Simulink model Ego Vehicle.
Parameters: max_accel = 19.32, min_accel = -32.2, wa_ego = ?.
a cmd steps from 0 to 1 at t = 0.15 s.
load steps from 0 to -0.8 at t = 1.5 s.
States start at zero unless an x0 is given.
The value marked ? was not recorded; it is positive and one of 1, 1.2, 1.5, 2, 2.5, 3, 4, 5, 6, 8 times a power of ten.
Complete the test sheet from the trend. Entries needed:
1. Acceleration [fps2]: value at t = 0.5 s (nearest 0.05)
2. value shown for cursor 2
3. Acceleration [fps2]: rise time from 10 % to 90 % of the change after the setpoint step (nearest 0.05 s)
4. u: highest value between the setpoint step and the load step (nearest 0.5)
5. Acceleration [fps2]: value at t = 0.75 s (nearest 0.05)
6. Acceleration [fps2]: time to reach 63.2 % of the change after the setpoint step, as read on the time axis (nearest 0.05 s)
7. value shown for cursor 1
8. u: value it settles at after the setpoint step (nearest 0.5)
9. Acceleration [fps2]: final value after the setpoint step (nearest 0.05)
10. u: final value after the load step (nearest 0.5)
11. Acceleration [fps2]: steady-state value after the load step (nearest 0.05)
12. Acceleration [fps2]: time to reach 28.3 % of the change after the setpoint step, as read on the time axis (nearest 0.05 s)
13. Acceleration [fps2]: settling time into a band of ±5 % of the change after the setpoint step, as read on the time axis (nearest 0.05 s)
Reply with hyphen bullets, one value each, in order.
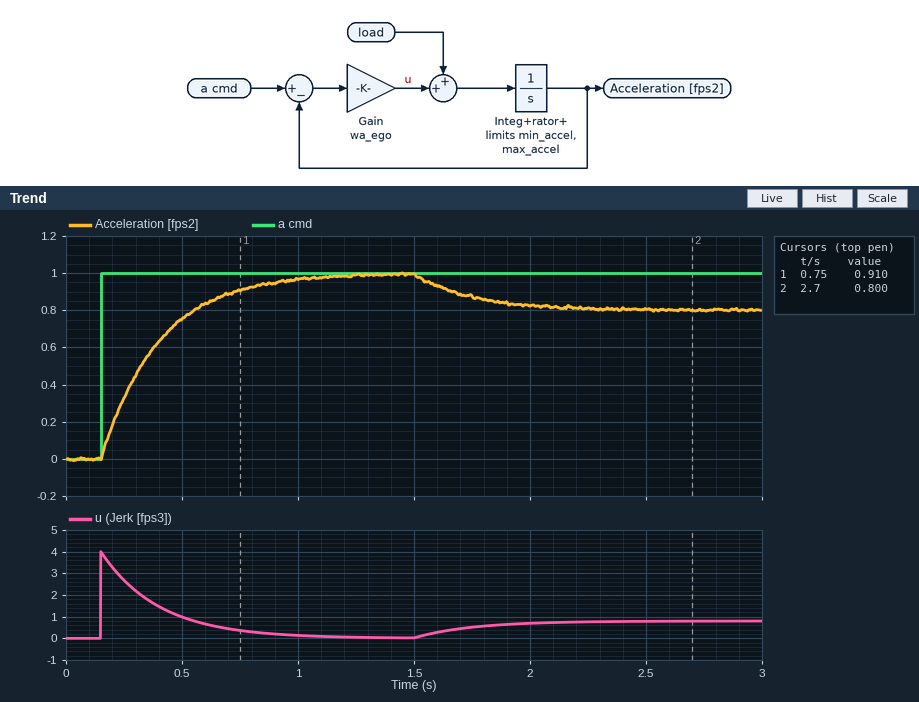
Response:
- 0.75
- 0.800
- 0.55 s
- 4.0
- 0.90
- 0.40 s
- 0.910
- 0.0
- 1.00
- 1.0
- 0.80
- 0.25 s
- 0.90 s
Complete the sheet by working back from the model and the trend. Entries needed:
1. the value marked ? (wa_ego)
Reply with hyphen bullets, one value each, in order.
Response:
- 4
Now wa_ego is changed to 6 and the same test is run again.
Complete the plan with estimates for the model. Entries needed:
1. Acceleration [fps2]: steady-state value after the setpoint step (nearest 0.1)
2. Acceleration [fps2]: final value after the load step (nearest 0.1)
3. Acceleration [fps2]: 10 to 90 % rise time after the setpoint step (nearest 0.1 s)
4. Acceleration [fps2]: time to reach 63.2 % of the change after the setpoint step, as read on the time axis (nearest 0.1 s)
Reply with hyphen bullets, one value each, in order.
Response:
- 1.0
- 0.9
- 0.4 s
- 0.3 s
